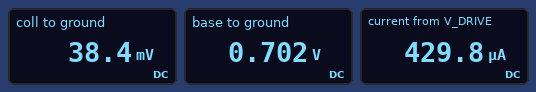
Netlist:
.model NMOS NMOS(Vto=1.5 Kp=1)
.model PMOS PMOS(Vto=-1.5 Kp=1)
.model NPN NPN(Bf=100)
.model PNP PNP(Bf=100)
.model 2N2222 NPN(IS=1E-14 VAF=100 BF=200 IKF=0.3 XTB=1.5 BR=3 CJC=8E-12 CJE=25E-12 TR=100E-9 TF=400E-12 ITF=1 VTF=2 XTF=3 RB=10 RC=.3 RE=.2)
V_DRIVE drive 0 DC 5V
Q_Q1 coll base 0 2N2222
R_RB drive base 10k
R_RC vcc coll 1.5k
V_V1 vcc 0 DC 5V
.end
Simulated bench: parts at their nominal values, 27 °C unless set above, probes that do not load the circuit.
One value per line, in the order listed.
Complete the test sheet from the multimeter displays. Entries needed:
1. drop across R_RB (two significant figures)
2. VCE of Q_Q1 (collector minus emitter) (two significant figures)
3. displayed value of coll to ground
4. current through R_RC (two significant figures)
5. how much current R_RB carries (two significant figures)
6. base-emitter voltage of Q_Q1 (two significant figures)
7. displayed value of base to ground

4.3 V
38 mV
38.4 mV
3.3 mA
430 µA
700 mV
0.702 V
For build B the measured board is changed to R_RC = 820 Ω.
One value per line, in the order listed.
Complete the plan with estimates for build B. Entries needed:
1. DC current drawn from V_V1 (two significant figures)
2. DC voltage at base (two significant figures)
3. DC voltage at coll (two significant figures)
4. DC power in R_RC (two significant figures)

6.0 mA
710 mV
52 mV
30 mW
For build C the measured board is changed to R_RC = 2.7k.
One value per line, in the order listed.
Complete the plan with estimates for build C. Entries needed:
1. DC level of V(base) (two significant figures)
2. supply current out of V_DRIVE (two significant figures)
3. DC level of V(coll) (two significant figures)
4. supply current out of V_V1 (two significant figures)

690 mV
430 µA
28 mV
1.8 mA
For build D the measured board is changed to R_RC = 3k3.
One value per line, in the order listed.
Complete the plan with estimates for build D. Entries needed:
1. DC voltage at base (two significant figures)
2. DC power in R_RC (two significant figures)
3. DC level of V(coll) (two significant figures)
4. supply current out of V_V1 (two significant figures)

690 mV
7.5 mW
25 mV
1.5 mA
